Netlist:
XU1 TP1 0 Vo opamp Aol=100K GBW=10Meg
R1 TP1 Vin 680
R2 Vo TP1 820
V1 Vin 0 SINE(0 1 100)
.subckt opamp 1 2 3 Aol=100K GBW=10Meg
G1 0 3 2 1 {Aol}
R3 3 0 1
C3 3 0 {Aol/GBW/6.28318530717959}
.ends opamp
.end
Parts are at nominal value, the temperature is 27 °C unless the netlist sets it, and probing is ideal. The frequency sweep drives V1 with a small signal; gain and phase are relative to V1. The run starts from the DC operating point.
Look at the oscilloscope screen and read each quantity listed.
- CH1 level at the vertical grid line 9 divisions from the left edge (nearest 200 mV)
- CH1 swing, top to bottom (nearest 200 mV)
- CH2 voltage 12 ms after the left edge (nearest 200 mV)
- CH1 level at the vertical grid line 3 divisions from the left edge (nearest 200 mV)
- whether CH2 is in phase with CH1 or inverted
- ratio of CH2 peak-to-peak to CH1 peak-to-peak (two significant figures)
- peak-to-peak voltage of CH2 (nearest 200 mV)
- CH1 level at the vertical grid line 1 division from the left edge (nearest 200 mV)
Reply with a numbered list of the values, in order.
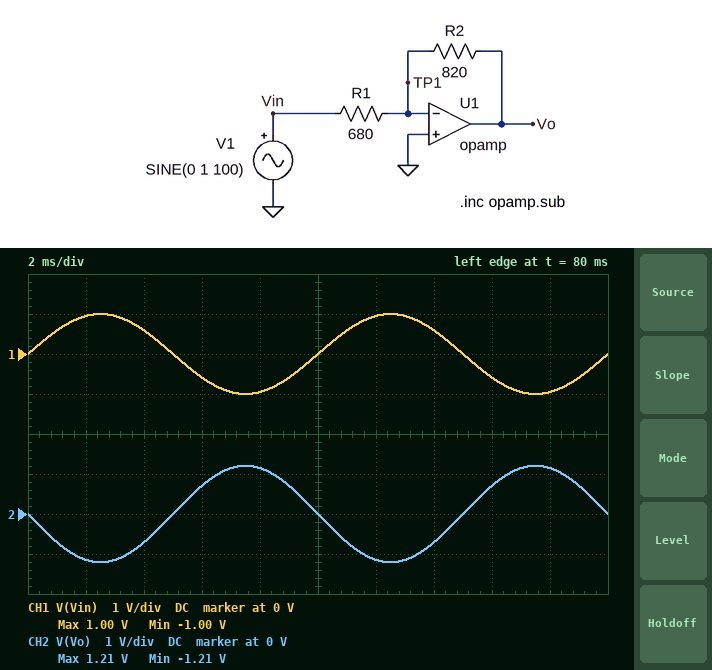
1. -1.0 V
2. 2.0 V
3. -1.2 V
4. -600 mV
5. inverted
6. 1.2
7. 2.4 V
8. 1.0 V
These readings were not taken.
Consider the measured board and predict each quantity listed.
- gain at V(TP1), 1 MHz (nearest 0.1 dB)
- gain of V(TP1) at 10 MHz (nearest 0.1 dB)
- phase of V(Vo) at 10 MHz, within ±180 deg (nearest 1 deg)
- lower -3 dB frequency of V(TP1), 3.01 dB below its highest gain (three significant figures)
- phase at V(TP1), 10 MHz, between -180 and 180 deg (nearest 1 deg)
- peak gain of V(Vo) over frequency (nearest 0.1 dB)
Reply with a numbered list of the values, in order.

1. -18.6 dB
2. -6.1 dB
3. 114 deg
4. 4.53 MHz
5. 24 deg
6. 1.6 dB
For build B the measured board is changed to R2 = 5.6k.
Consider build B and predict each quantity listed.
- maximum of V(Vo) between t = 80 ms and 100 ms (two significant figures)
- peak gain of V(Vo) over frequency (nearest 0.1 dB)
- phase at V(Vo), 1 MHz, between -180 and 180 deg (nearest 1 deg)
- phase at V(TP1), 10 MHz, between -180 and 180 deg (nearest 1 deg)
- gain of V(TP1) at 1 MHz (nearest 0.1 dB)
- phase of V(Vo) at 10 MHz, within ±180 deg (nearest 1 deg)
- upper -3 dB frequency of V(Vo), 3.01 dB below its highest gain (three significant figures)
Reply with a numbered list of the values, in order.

1. 8.2 V
2. 18.3 dB
3. 137 deg
4. 6 deg
5. -4.4 dB
6. 96 deg
7. 1.08 MHz
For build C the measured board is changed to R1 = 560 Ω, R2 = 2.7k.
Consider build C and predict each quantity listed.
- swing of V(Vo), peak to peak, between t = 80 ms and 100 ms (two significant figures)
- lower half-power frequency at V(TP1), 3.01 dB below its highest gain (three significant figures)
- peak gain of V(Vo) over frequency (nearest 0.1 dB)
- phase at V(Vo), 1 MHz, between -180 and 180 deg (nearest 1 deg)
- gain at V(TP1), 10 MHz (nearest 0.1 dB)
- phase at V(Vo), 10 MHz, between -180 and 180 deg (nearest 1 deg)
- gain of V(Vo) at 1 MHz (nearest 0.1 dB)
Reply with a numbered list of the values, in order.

1. 9.6 V
2. 1.72 MHz
3. 13.7 dB
4. 150 deg
5. -1.8 dB
6. 100 deg
7. 12.4 dB
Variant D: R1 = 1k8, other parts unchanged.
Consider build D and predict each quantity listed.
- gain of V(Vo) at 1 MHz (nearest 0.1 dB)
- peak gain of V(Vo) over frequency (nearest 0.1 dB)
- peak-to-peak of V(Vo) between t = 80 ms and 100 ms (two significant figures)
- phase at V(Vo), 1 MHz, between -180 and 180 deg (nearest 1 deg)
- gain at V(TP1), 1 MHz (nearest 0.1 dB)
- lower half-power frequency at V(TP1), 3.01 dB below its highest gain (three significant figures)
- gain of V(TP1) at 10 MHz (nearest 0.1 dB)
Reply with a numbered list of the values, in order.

1. -6.9 dB
2. -6.8 dB
3. 910 mV
4. 172 deg
5. -26.9 dB
6. 6.87 MHz
7. -11.8 dB
